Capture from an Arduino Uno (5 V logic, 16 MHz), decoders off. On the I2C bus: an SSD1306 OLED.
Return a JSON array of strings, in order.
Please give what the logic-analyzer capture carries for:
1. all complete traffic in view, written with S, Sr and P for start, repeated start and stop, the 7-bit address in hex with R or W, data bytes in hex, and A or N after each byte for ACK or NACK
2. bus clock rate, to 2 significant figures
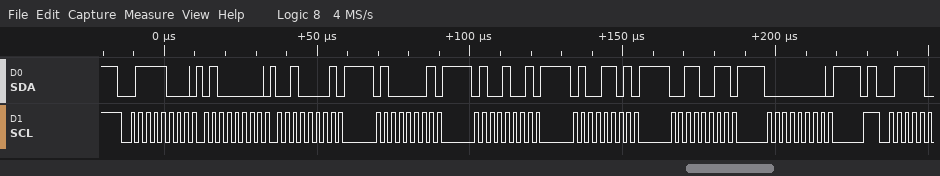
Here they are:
["S 3CW A 40 A 21 A 41 A 49 A 4D A 33 A 00 A P", "400 kHz"]
